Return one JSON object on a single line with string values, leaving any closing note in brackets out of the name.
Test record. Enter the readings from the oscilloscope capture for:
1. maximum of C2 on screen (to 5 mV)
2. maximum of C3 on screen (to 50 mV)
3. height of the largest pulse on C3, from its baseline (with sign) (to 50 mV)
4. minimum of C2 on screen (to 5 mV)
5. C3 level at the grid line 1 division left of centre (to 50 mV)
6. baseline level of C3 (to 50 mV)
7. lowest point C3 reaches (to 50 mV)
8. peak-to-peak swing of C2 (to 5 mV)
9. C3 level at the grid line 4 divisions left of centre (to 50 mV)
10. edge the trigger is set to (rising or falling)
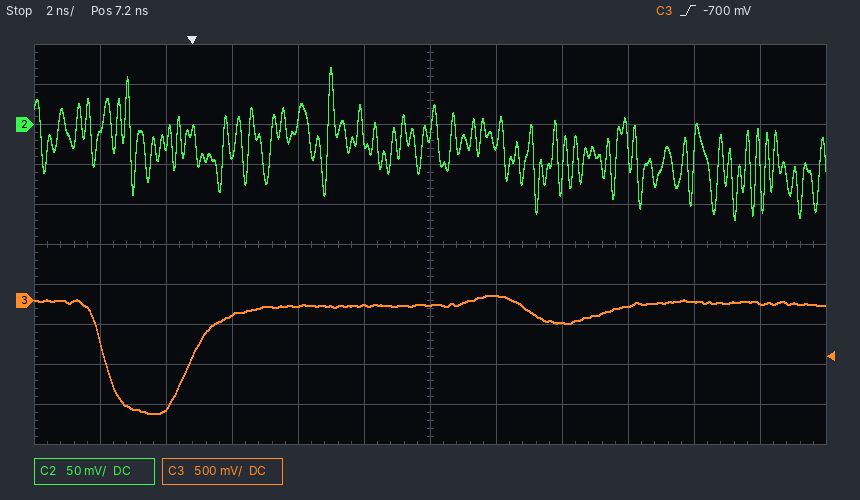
{"maximum of C2 on screen": "70 mV", "maximum of C3 on screen": "50 mV", "height of the largest pulse on C3, from its baseline (with sign)": "-1.35 V", "minimum of C2 on screen": "-120 mV", "C3 level at the grid line 1 division left of centre": "-50 mV", "baseline level of C3": "-50 mV", "lowest point C3 reaches": "-1.40 V", "peak-to-peak swing of C2": "190 mV", "C3 level at the grid line 4 divisions left of centre": "-1.35 V", "edge the trigger is set to": "rising"}
